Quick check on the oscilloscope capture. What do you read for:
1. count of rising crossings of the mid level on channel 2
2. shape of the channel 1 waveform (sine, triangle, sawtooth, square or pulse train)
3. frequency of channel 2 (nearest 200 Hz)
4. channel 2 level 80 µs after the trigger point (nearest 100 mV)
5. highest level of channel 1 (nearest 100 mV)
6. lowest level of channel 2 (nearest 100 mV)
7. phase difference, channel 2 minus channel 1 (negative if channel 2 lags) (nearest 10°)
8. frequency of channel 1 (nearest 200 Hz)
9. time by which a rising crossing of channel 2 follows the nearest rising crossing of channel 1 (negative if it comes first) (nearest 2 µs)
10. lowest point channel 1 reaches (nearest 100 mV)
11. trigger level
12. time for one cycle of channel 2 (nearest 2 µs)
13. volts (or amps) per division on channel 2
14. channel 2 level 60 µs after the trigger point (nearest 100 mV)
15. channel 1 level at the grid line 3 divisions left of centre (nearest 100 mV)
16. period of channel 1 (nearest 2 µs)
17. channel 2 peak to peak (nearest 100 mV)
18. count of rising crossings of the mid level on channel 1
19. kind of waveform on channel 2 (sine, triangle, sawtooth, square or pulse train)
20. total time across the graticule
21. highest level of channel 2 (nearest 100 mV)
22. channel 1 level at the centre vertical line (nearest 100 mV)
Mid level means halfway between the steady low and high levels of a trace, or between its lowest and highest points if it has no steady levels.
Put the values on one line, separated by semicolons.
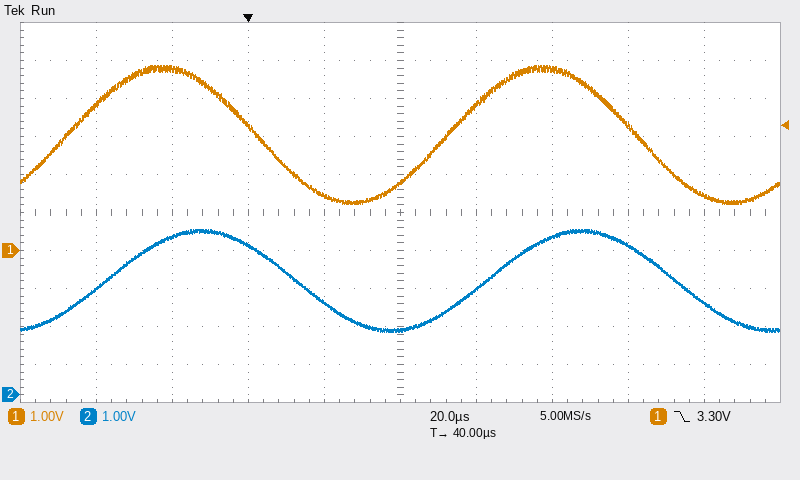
2; sine; 10.0 kHz; 4.2 V; 4.9 V; 1.7 V; -40°; 10.0 kHz; +10 µs; 1.2 V; 3.30 V; 100 µs; 1 V; 2.8 V; 4.8 V; 100 µs; 2.7 V; 2; sine; 200 µs; 4.4 V; 1.8 V
